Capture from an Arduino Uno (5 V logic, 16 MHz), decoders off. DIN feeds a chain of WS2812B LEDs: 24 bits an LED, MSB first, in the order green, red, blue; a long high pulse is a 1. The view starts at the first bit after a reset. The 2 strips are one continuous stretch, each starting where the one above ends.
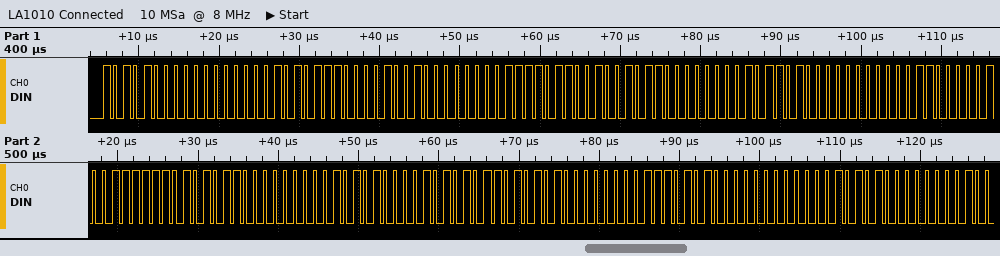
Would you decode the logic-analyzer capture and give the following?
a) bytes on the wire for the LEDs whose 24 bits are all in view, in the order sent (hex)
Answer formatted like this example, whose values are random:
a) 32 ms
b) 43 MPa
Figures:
a) A8 00 57 09 00 F6 4B 00 B4 00 60 9F AB 00 54 2A D5 00 EA 00 15
